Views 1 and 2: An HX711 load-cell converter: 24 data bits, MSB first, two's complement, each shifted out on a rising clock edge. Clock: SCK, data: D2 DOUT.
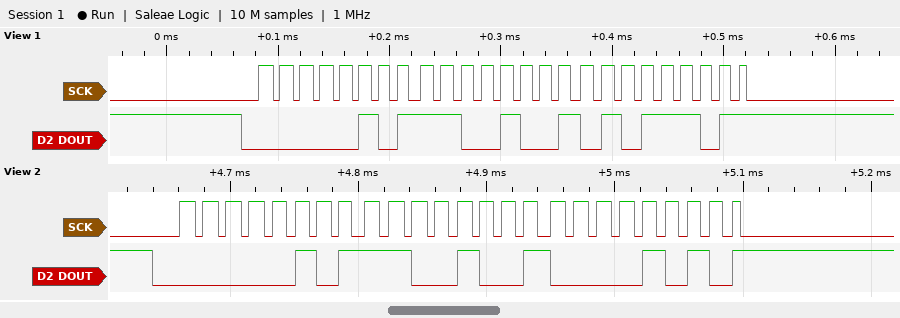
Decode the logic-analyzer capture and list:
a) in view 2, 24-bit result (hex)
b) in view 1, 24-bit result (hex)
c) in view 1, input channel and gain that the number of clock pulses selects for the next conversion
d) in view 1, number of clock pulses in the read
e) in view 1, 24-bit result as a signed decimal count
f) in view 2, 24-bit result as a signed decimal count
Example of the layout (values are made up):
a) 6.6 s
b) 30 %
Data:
a) 0x05C90A
b) 0x05C95D
c) channel A, gain 128
d) 25
e) 379229
f) 379146
